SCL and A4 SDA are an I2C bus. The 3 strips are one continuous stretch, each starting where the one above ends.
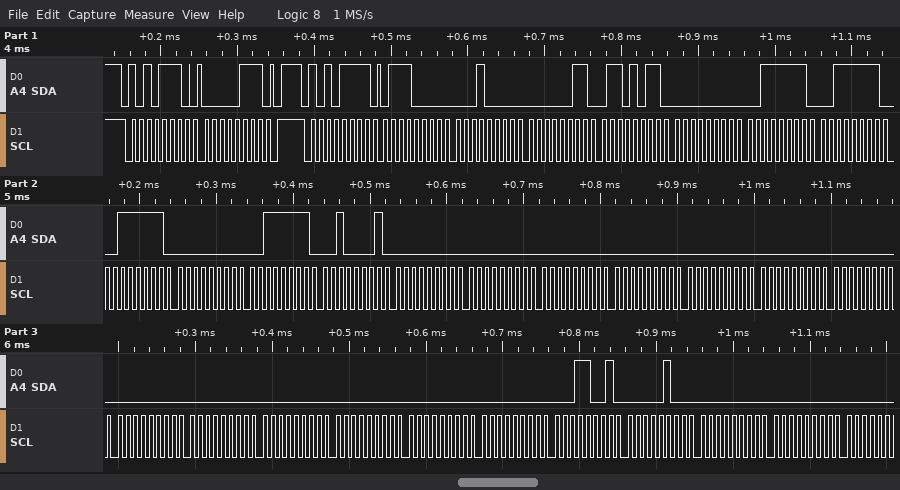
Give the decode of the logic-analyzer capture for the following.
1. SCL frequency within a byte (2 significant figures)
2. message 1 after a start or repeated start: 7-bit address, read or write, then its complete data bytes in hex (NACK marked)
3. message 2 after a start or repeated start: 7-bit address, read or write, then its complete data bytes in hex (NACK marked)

100 kHz
0x57 write: 07
0x57 read: 70 10 03 6B 00 3F 3F 3F 00 3F 21 00 00 00 00 00 00 00 00 00 00 00 00 00 19 04 00 00
